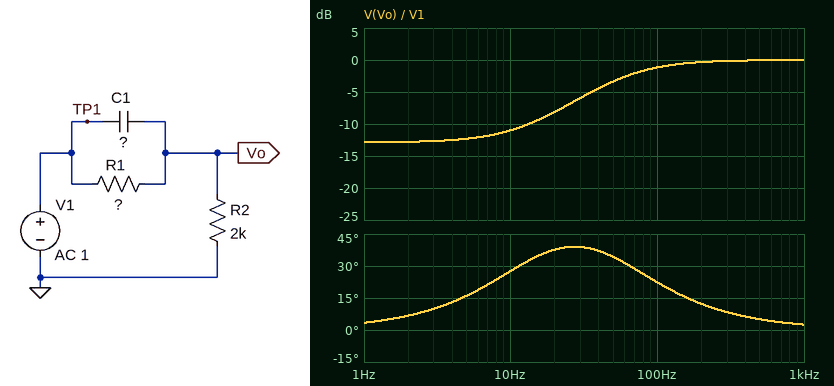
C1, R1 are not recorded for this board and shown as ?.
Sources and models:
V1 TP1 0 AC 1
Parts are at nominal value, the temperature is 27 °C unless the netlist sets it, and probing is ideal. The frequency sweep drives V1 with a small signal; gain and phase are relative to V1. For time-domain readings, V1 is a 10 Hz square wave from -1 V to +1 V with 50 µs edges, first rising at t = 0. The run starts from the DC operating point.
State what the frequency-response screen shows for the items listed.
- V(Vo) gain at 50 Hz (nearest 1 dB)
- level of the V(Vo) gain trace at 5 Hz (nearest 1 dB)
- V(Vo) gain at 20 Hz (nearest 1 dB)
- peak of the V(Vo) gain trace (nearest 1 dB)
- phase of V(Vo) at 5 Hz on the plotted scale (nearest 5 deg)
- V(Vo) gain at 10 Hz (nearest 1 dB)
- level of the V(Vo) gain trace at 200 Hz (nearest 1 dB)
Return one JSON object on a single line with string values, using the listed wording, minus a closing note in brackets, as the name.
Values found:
{"V(Vo) gain at 50 Hz": "-3 dB", "level of the V(Vo) gain trace at 5 Hz": "-12 dB", "V(Vo) gain at 20 Hz": "-8 dB", "peak of the V(Vo) gain trace": "0 dB", "phase of V(Vo) at 5 Hz on the plotted scale": "15 deg", "V(Vo) gain at 10 Hz": "-11 dB", "level of the V(Vo) gain trace at 200 Hz": "0 dB"}
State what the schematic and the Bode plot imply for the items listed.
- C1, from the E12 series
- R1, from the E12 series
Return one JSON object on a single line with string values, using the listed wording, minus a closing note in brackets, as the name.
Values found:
{"C1, from the E12 series": "1.8 µF", "R1, from the E12 series": "6.8 kΩ"}
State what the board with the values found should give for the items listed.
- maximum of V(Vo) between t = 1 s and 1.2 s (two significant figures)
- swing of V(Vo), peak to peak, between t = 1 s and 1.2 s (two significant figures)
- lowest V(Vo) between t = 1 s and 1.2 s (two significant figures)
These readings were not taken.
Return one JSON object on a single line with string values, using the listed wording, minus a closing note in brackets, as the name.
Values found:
{"maximum of V(Vo) between t = 1 s and 1.2 s": "1.8 V", "swing of V(Vo), peak to peak, between t = 1 s and 1.2 s": "3.5 V", "lowest V(Vo) between t = 1 s and 1.2 s": "-1.8 V"}
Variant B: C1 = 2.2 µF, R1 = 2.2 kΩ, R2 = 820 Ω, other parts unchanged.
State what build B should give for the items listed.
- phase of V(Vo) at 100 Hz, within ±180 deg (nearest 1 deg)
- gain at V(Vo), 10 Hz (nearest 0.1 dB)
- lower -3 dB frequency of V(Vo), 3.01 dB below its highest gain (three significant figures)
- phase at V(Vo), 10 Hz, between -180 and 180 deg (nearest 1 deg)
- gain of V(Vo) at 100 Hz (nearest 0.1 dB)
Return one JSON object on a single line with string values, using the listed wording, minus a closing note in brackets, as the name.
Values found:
{"phase of V(Vo) at 100 Hz, within ±180 deg": "32 deg", "gain at V(Vo), 10 Hz": "-11.0 dB", "lower -3 dB frequency of V(Vo), 3.01 dB below its highest gain": "112 Hz", "phase at V(Vo), 10 Hz, between -180 and 180 deg": "12 deg", "gain of V(Vo) at 100 Hz": "-3.5 dB"}
